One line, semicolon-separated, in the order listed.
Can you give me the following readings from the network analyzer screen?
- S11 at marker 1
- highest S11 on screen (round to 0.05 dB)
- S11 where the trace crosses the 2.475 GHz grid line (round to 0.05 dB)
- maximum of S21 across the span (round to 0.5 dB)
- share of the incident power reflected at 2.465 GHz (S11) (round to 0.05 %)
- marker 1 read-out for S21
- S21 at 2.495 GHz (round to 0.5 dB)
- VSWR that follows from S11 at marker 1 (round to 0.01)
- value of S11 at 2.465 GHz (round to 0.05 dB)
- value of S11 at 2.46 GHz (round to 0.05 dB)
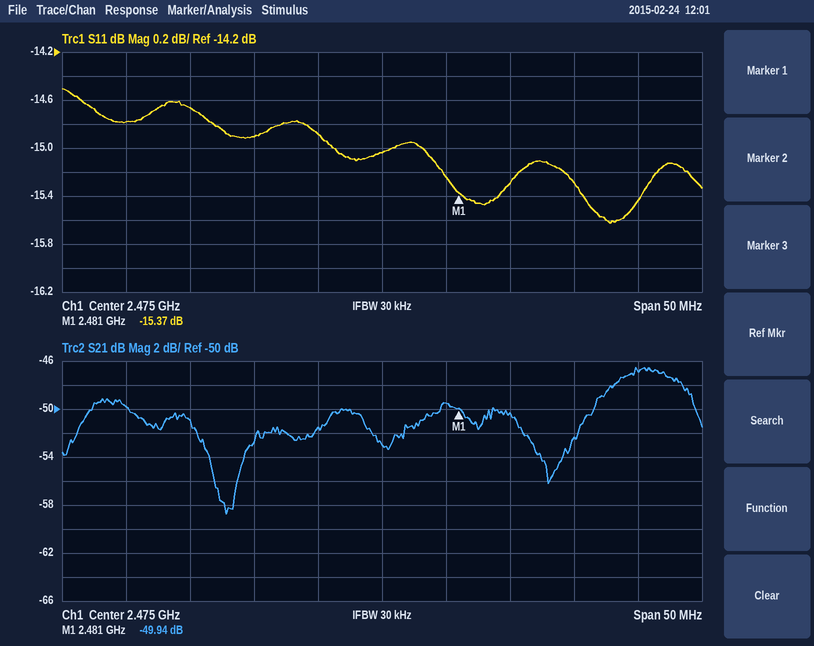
-15.37 dB; -14.50 dB; -15.05 dB; -46.5 dB; 3.25 %; -49.94 dB; -47.0 dB; 1.41; -14.90 dB; -14.65 dB
